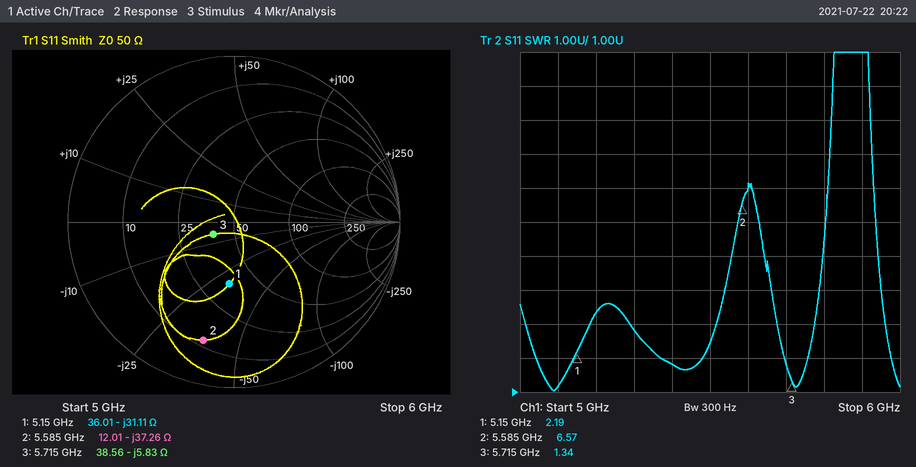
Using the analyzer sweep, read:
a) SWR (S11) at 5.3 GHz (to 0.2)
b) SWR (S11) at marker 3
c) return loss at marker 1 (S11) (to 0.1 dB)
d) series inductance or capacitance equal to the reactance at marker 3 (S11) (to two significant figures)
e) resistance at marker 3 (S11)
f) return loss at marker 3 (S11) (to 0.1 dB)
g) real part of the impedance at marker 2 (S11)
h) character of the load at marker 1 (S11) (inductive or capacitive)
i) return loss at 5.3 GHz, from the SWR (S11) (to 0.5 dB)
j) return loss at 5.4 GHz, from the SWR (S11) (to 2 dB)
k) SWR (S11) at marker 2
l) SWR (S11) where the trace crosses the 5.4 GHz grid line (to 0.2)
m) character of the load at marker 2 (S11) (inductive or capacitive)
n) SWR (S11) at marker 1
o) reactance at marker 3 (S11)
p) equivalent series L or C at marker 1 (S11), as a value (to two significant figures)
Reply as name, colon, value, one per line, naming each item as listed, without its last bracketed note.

SWR (S11) at 5.3 GHz: 2.8
SWR (S11) at marker 3: 1.34
return loss at marker 1 (S11): 8.6 dB
series inductance or capacitance equal to the reactance at marker 3 (S11): 4.8 pF
resistance at marker 3: 38.56 Ω
return loss at marker 3 (S11): 16.8 dB
real part of the impedance at marker 2: 12.01 Ω
character of the load at marker 1 (S11): capacitive
return loss at 5.3 GHz, from the SWR (S11): 6.5 dB
return loss at 5.4 GHz, from the SWR (S11): 10 dB
SWR (S11) at marker 2: 6.57
SWR (S11) where the trace crosses the 5.4 GHz grid line: 1.8
character of the load at marker 2 (S11): capacitive
SWR (S11) at marker 1: 2.19
reactance at marker 3: -5.83 Ω
equivalent series L or C at marker 1 (S11), as a value: 990 fF
